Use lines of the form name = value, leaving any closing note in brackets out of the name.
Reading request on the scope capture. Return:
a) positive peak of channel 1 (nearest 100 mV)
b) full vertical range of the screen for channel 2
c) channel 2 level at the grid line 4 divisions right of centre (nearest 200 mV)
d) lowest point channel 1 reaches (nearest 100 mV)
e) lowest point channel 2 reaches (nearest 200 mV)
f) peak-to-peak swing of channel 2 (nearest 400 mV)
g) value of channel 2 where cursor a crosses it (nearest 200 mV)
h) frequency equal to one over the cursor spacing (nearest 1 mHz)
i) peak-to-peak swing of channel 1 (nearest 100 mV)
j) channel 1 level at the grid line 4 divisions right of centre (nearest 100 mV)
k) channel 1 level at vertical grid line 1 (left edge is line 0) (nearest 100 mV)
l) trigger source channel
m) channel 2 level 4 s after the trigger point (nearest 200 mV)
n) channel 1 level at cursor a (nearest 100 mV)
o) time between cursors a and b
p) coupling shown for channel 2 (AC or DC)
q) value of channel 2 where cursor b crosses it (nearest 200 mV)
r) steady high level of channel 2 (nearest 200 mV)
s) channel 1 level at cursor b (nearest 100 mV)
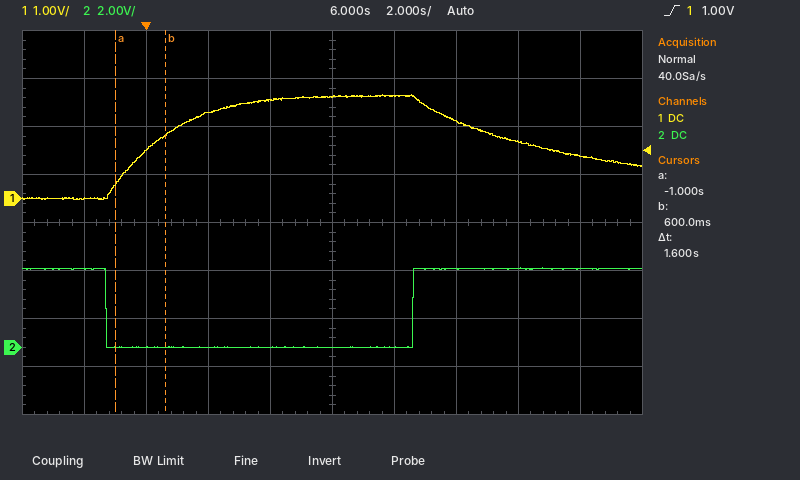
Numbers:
positive peak of channel 1 = 2.2 V
full vertical range of the screen for channel 2 = 16 V
channel 2 level at the grid line 4 divisions right of centre = 3.2 V
lowest point channel 1 reaches = 0.0 V
lowest point channel 2 reaches = 0.0 V
peak-to-peak swing of channel 2 = 3.2 V
value of channel 2 where cursor a crosses it = 0.0 V
frequency equal to one over the cursor spacing = 625 mHz
peak-to-peak swing of channel 1 = 2.2 V
channel 1 level at the grid line 4 divisions right of centre = 900 mV
channel 1 level at vertical grid line 1 (left edge is line 0) = 0.0 V
trigger source channel = channel 1
channel 2 level 4 s after the trigger point = 0.0 V
channel 1 level at cursor a = 300 mV
time between cursors a and b = 1.6 s
coupling shown for channel 2 = DC
value of channel 2 where cursor b crosses it = 0.0 V
steady high level of channel 2 = 3.2 V
channel 1 level at cursor b = 1.3 V
